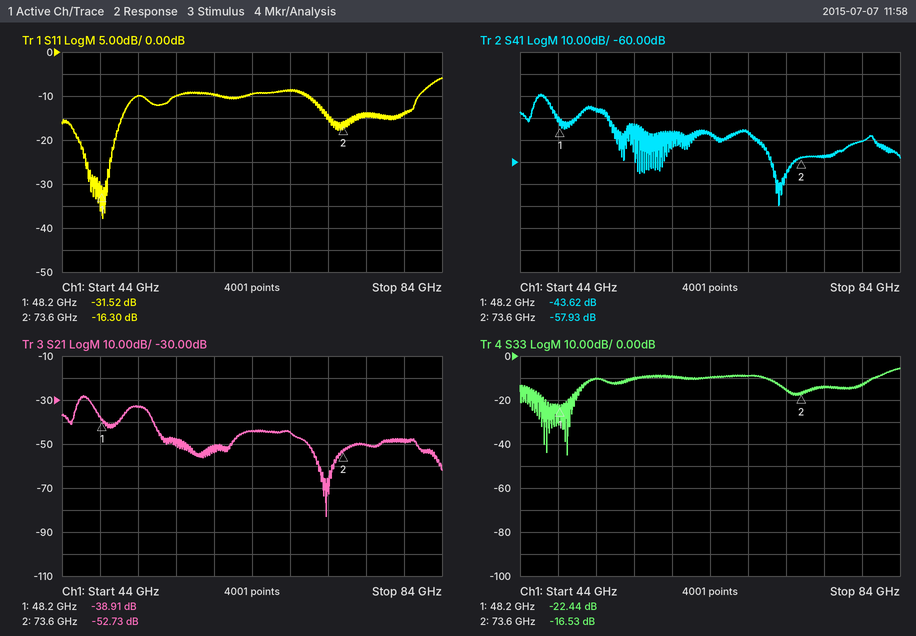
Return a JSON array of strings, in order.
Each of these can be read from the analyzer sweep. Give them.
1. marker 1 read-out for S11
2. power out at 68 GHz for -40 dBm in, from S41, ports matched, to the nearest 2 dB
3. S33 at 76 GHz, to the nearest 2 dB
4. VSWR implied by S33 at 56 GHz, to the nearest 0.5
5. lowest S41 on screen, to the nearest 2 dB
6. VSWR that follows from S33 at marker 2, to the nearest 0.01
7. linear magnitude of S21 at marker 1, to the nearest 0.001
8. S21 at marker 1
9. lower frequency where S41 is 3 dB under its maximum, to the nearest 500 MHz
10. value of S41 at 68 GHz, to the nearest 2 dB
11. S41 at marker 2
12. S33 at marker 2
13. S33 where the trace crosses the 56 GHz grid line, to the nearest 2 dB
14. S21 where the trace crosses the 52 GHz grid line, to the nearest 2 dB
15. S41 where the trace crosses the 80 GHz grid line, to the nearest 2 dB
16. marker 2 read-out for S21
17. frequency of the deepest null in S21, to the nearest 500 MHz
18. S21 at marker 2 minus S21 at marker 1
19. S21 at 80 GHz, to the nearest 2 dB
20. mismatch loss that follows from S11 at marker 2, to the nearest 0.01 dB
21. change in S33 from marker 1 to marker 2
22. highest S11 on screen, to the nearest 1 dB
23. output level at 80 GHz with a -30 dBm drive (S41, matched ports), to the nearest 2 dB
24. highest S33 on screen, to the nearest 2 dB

["-31.52 dB", "-86 dBm", "-14 dB", "2.0", "-80 dB", "1.35", "0.011", "-38.91 dB", "45.5 GHz", "-46 dB", "-57.93 dB", "-16.53 dB", "-10 dB", "-32 dB", "-50 dB", "-52.73 dB", "72.0 GHz", "-13.82 dB", "-48 dB", "0.10 dB", "5.91 dB", "-6 dB", "-80 dBm", "-6 dB"]
